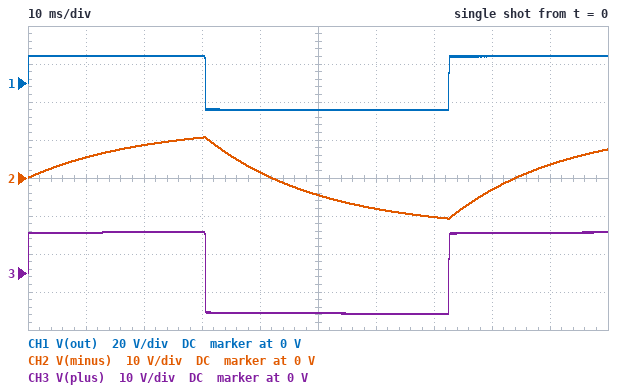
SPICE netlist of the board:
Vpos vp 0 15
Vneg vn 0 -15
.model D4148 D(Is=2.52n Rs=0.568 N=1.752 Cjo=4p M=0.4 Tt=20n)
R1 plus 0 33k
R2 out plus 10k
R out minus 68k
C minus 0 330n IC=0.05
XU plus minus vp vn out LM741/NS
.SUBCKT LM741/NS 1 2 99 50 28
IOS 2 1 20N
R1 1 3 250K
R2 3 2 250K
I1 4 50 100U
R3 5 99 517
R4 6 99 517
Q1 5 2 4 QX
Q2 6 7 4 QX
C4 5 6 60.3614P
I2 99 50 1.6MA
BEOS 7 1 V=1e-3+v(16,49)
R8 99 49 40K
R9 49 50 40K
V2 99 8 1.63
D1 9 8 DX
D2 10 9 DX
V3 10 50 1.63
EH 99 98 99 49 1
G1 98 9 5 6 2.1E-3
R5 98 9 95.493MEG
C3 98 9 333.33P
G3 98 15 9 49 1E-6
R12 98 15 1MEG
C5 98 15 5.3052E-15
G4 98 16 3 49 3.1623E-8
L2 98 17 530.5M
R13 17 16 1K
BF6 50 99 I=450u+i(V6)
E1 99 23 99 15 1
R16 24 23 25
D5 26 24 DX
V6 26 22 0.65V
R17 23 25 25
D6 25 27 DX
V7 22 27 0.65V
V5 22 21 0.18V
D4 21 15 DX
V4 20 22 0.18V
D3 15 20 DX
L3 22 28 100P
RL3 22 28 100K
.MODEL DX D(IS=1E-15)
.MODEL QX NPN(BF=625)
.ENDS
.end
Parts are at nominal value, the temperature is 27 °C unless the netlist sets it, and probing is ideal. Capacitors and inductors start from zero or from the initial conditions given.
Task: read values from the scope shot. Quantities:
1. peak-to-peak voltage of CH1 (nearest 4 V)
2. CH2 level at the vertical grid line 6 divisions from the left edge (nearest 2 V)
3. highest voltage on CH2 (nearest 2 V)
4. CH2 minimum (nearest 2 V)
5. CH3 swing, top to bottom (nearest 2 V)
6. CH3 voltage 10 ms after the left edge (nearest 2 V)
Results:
28 V
-8 V
10 V
-10 V
22 V
10 V
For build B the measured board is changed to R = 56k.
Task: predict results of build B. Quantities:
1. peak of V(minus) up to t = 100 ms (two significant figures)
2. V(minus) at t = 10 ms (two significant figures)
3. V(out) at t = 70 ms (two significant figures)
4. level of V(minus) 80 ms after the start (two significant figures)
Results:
11 V
6.2 V
14 V
6.1 V
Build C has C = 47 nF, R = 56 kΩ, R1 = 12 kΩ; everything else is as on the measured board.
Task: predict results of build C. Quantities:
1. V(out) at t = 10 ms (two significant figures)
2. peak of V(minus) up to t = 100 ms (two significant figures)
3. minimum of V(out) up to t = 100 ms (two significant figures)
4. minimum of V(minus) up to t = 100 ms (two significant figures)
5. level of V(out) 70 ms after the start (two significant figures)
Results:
-14 V
7.6 V
-14 V
-7.6 V
14 V
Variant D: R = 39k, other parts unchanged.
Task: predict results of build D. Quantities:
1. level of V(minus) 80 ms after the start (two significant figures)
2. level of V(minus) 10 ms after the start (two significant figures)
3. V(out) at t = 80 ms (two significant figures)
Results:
-4.9 V
7.8 V
-14 V
